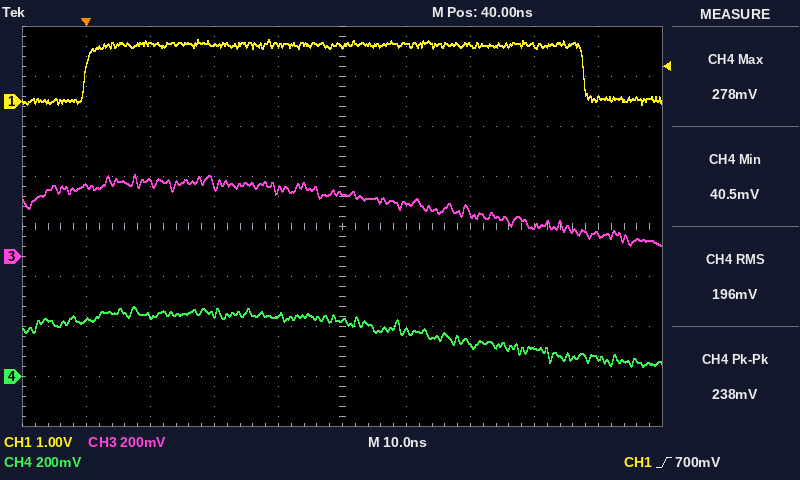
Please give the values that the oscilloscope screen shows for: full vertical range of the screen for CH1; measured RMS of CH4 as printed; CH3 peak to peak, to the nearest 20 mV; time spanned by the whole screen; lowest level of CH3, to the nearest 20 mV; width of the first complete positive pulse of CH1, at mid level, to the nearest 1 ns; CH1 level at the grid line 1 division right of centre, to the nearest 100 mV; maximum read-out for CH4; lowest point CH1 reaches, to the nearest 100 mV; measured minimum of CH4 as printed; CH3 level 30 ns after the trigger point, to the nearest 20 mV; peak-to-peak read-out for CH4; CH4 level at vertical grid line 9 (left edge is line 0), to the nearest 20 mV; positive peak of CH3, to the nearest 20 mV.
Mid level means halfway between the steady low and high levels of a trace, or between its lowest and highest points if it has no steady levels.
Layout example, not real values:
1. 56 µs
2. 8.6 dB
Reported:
1. 8 V
2. 196 mV
3. 280 mV
4. 100 ns
5. 40 mV
6. 78 ns
7. 1.2 V
8. 278 mV
9. -100 mV
10. 40.5 mV
11. 260 mV
12. 238 mV
13. 80 mV
14. 320 mV
